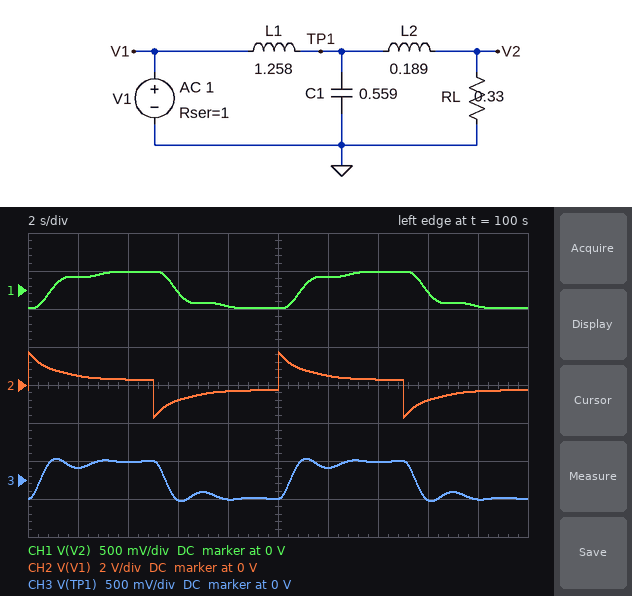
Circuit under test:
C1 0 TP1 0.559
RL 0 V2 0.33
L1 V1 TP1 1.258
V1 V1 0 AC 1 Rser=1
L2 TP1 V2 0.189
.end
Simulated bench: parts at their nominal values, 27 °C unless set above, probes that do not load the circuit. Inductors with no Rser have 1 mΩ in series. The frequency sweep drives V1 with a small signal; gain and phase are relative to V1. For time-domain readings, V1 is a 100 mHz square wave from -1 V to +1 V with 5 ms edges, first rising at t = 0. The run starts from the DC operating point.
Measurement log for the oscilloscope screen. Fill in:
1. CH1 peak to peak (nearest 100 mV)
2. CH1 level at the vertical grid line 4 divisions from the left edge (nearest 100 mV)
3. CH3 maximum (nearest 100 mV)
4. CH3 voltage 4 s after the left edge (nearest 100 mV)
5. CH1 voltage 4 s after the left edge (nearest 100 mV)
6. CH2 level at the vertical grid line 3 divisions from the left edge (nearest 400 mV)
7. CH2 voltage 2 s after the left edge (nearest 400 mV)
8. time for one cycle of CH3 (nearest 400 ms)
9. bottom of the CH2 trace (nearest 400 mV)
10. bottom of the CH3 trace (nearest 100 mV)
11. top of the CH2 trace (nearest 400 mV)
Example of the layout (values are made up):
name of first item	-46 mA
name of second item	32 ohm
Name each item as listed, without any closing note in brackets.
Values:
CH1 peak to peak	500 mV
CH1 level at the vertical grid line 4 divisions from the left edge	-200 mV
CH3 maximum	300 mV
CH3 voltage 4 s after the left edge	200 mV
CH1 voltage 4 s after the left edge	200 mV
CH2 level at the vertical grid line 3 divisions from the left edge	-800 mV
CH2 voltage 2 s after the left edge	400 mV
time for one cycle of CH3	10.0 s
bottom of the CH2 trace	-1.6 V
bottom of the CH3 trace	-300 mV
top of the CH2 trace	1.6 V
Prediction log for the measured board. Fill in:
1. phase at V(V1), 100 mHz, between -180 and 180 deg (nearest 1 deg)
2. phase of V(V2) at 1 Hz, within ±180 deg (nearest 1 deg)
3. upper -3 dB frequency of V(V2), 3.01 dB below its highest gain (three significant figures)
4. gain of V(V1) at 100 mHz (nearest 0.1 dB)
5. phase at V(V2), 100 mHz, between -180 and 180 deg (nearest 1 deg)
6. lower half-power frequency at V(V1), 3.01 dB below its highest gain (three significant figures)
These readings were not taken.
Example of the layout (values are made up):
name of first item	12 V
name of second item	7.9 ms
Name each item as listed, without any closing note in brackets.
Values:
phase at V(V1), 100 mHz, between -180 and 180 deg	35 deg
phase of V(V2) at 1 Hz, within ±180 deg	118 deg
upper -3 dB frequency of V(V2), 3.01 dB below its highest gain	180 mHz
gain of V(V1) at 100 mHz	-4.7 dB
phase at V(V2), 100 mHz, between -180 and 180 deg	-40 deg
lower half-power frequency at V(V1), 3.01 dB below its highest gain	146 mHz
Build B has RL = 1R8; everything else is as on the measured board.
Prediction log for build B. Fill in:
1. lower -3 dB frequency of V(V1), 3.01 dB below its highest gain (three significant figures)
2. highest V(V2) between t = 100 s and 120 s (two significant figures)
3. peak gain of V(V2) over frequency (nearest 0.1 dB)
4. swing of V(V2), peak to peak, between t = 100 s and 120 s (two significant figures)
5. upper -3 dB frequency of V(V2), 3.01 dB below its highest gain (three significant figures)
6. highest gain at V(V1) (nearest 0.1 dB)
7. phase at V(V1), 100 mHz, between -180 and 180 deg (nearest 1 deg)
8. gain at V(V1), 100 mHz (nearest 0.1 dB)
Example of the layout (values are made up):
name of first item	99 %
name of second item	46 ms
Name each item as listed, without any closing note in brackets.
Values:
lower -3 dB frequency of V(V1), 3.01 dB below its highest gain	274 mHz
highest V(V2) between t = 100 s and 120 s	760 mV
peak gain of V(V2) over frequency	-3.5 dB
swing of V(V2), peak to peak, between t = 100 s and 120 s	1.5 V
upper -3 dB frequency of V(V2), 3.01 dB below its highest gain	277 mHz
highest gain at V(V1)	0 dB
phase at V(V1), 100 mHz, between -180 and 180 deg	0 deg
gain at V(V1), 100 mHz	-4.8 dB
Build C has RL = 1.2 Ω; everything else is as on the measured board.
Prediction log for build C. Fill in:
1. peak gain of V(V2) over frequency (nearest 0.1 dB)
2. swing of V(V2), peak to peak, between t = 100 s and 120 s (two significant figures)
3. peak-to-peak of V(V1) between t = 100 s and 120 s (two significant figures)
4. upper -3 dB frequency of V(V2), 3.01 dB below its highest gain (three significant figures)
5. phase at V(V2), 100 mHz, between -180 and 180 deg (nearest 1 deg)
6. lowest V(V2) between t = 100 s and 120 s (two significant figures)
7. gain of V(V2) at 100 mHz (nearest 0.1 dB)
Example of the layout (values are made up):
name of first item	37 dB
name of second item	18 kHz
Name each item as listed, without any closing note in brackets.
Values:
peak gain of V(V2) over frequency	-5.3 dB
swing of V(V2), peak to peak, between t = 100 s and 120 s	1.2 V
peak-to-peak of V(V1) between t = 100 s and 120 s	2.9 V
upper -3 dB frequency of V(V2), 3.01 dB below its highest gain	282 mHz
phase at V(V2), 100 mHz, between -180 and 180 deg	-35 deg
lowest V(V2) between t = 100 s and 120 s	-580 mV
gain of V(V2) at 100 mHz	-5.4 dB
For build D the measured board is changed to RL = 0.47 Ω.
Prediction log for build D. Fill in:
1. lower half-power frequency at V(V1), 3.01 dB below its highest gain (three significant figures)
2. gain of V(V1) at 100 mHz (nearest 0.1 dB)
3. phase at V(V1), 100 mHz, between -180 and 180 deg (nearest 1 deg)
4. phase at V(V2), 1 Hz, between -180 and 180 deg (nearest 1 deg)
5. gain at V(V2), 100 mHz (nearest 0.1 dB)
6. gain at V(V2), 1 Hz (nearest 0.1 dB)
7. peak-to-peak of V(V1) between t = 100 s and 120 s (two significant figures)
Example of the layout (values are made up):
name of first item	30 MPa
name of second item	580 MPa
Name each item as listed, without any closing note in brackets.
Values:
lower half-power frequency at V(V1), 3.01 dB below its highest gain	163 mHz
gain of V(V1) at 100 mHz	-5.0 dB
phase at V(V1), 100 mHz, between -180 and 180 deg	30 deg
phase at V(V2), 1 Hz, between -180 and 180 deg	125 deg
gain at V(V2), 100 mHz	-11.0 dB
gain at V(V2), 1 Hz	-35.3 dB
peak-to-peak of V(V1) between t = 100 s and 120 s	3.3 V
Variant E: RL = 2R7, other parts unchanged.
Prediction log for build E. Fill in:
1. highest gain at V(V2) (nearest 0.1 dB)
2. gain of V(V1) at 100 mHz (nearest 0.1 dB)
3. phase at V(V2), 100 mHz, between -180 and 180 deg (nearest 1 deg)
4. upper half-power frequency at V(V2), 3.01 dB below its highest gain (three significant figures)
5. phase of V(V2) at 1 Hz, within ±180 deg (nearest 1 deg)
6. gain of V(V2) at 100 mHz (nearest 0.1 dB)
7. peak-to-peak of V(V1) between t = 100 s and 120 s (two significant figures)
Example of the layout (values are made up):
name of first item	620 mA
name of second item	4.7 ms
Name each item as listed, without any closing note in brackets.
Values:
highest gain at V(V2)	-1.7 dB
gain of V(V1) at 100 mHz	-4.1 dB
phase at V(V2), 100 mHz, between -180 and 180 deg	-32 deg
upper half-power frequency at V(V2), 3.01 dB below its highest gain	264 mHz
phase of V(V2) at 1 Hz, within ±180 deg	169 deg
gain of V(V2) at 100 mHz	-2.1 dB
peak-to-peak of V(V1) between t = 100 s and 120 s	2.5 V
